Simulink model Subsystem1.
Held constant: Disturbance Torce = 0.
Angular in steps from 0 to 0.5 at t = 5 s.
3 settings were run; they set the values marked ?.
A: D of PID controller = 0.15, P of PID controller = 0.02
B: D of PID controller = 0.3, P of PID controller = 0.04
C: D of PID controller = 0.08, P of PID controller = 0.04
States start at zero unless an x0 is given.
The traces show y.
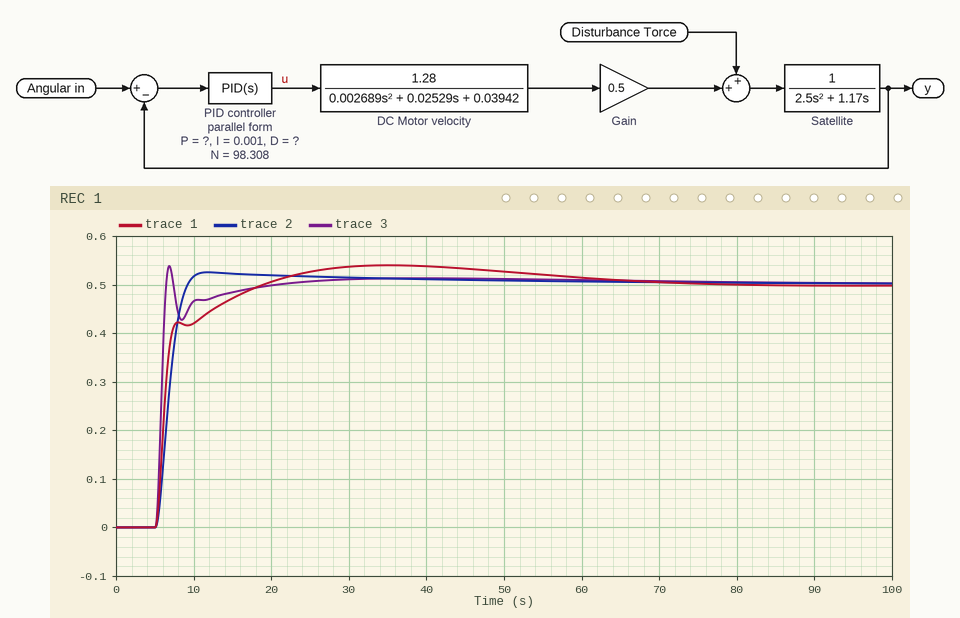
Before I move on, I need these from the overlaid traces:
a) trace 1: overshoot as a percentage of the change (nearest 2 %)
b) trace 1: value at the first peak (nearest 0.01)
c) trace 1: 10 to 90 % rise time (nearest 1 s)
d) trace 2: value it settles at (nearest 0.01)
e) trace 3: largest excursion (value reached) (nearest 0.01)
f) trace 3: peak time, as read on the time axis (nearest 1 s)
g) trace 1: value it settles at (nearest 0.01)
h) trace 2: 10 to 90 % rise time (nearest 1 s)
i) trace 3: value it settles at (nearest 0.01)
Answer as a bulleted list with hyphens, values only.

- 8 %
- 0.54
- 7 s
- 0.50
- 0.54
- 7 s
- 0.50
- 3 s
- 0.50
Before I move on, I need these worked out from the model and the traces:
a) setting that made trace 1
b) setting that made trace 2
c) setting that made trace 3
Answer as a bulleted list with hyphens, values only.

- A
- C
- B
